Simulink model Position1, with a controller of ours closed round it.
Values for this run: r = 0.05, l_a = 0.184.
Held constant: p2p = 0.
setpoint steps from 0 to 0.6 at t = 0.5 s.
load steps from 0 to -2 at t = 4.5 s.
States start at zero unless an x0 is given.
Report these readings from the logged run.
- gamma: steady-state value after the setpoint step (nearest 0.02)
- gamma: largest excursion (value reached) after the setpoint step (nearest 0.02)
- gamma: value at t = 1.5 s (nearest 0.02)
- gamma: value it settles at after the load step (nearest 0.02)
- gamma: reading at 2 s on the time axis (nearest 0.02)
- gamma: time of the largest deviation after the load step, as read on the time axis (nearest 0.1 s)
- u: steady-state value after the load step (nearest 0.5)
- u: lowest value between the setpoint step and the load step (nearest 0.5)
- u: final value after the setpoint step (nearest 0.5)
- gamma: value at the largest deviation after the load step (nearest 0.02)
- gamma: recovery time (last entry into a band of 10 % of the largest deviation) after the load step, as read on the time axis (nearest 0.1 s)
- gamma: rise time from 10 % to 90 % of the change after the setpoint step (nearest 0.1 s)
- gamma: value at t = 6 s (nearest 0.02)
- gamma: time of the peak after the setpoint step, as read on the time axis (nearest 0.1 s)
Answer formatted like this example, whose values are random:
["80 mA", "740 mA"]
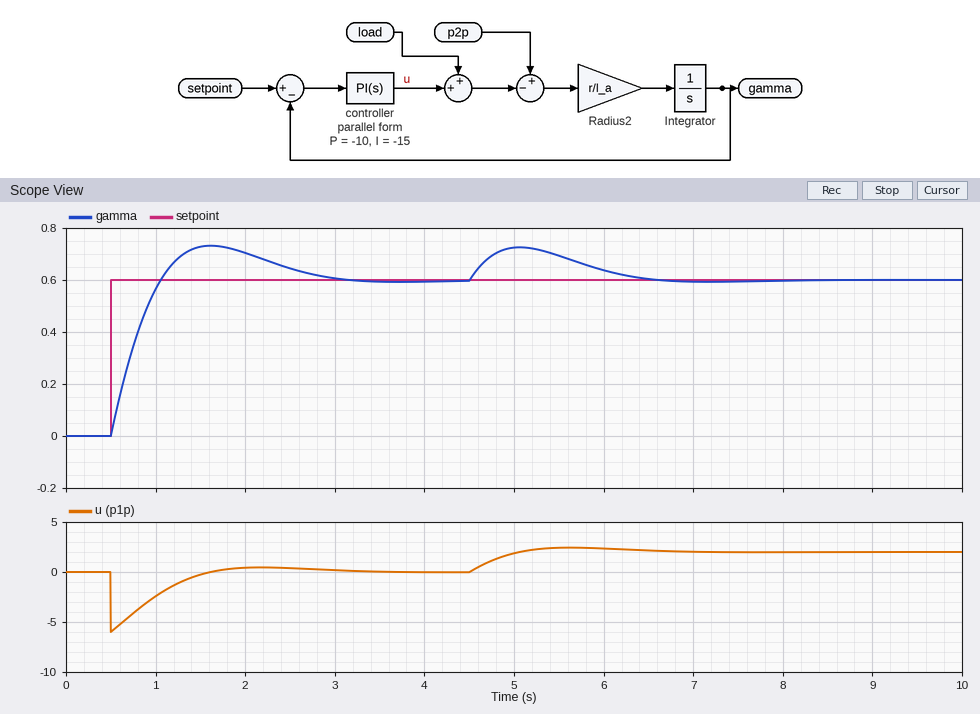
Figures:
["0.60", "0.74", "0.72", "0.60", "0.70", "5.1 s", "2.0", "-6.0", "0.0", "0.72", "6.3 s", "0.4 s", "0.64", "1.6 s"]
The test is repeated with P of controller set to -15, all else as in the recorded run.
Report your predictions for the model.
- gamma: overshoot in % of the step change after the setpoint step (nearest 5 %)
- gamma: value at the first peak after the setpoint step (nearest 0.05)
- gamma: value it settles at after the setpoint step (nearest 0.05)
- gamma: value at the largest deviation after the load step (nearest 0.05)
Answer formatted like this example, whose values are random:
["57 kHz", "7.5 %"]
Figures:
["15 %", "0.70", "0.60", "0.70"]
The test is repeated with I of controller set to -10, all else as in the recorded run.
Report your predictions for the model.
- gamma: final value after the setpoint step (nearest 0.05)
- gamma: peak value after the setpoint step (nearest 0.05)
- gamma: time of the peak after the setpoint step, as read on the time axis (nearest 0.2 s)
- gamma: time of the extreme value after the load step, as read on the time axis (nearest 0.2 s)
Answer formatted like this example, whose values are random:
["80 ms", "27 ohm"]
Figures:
["0.60", "0.70", "1.8 s", "5.2 s"]
